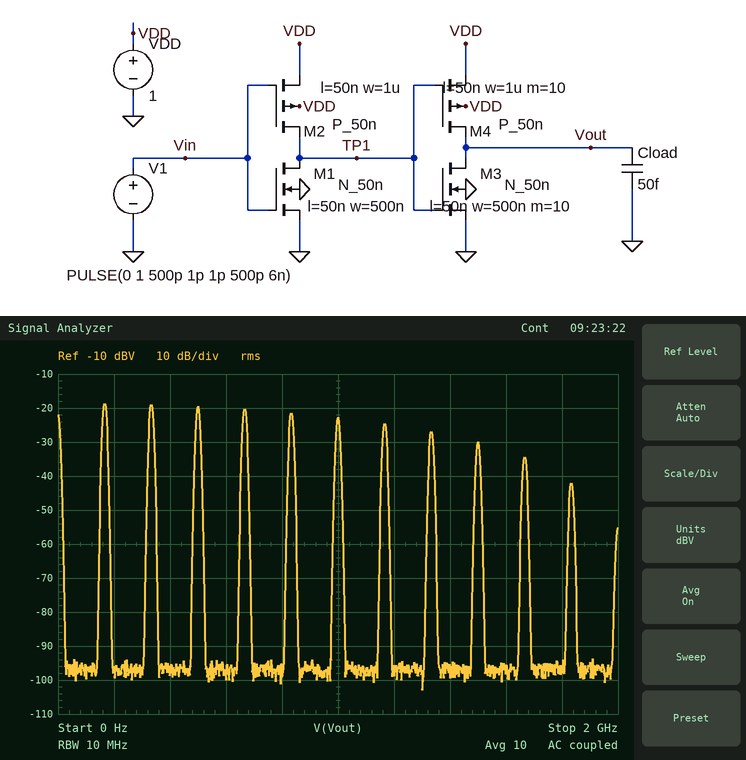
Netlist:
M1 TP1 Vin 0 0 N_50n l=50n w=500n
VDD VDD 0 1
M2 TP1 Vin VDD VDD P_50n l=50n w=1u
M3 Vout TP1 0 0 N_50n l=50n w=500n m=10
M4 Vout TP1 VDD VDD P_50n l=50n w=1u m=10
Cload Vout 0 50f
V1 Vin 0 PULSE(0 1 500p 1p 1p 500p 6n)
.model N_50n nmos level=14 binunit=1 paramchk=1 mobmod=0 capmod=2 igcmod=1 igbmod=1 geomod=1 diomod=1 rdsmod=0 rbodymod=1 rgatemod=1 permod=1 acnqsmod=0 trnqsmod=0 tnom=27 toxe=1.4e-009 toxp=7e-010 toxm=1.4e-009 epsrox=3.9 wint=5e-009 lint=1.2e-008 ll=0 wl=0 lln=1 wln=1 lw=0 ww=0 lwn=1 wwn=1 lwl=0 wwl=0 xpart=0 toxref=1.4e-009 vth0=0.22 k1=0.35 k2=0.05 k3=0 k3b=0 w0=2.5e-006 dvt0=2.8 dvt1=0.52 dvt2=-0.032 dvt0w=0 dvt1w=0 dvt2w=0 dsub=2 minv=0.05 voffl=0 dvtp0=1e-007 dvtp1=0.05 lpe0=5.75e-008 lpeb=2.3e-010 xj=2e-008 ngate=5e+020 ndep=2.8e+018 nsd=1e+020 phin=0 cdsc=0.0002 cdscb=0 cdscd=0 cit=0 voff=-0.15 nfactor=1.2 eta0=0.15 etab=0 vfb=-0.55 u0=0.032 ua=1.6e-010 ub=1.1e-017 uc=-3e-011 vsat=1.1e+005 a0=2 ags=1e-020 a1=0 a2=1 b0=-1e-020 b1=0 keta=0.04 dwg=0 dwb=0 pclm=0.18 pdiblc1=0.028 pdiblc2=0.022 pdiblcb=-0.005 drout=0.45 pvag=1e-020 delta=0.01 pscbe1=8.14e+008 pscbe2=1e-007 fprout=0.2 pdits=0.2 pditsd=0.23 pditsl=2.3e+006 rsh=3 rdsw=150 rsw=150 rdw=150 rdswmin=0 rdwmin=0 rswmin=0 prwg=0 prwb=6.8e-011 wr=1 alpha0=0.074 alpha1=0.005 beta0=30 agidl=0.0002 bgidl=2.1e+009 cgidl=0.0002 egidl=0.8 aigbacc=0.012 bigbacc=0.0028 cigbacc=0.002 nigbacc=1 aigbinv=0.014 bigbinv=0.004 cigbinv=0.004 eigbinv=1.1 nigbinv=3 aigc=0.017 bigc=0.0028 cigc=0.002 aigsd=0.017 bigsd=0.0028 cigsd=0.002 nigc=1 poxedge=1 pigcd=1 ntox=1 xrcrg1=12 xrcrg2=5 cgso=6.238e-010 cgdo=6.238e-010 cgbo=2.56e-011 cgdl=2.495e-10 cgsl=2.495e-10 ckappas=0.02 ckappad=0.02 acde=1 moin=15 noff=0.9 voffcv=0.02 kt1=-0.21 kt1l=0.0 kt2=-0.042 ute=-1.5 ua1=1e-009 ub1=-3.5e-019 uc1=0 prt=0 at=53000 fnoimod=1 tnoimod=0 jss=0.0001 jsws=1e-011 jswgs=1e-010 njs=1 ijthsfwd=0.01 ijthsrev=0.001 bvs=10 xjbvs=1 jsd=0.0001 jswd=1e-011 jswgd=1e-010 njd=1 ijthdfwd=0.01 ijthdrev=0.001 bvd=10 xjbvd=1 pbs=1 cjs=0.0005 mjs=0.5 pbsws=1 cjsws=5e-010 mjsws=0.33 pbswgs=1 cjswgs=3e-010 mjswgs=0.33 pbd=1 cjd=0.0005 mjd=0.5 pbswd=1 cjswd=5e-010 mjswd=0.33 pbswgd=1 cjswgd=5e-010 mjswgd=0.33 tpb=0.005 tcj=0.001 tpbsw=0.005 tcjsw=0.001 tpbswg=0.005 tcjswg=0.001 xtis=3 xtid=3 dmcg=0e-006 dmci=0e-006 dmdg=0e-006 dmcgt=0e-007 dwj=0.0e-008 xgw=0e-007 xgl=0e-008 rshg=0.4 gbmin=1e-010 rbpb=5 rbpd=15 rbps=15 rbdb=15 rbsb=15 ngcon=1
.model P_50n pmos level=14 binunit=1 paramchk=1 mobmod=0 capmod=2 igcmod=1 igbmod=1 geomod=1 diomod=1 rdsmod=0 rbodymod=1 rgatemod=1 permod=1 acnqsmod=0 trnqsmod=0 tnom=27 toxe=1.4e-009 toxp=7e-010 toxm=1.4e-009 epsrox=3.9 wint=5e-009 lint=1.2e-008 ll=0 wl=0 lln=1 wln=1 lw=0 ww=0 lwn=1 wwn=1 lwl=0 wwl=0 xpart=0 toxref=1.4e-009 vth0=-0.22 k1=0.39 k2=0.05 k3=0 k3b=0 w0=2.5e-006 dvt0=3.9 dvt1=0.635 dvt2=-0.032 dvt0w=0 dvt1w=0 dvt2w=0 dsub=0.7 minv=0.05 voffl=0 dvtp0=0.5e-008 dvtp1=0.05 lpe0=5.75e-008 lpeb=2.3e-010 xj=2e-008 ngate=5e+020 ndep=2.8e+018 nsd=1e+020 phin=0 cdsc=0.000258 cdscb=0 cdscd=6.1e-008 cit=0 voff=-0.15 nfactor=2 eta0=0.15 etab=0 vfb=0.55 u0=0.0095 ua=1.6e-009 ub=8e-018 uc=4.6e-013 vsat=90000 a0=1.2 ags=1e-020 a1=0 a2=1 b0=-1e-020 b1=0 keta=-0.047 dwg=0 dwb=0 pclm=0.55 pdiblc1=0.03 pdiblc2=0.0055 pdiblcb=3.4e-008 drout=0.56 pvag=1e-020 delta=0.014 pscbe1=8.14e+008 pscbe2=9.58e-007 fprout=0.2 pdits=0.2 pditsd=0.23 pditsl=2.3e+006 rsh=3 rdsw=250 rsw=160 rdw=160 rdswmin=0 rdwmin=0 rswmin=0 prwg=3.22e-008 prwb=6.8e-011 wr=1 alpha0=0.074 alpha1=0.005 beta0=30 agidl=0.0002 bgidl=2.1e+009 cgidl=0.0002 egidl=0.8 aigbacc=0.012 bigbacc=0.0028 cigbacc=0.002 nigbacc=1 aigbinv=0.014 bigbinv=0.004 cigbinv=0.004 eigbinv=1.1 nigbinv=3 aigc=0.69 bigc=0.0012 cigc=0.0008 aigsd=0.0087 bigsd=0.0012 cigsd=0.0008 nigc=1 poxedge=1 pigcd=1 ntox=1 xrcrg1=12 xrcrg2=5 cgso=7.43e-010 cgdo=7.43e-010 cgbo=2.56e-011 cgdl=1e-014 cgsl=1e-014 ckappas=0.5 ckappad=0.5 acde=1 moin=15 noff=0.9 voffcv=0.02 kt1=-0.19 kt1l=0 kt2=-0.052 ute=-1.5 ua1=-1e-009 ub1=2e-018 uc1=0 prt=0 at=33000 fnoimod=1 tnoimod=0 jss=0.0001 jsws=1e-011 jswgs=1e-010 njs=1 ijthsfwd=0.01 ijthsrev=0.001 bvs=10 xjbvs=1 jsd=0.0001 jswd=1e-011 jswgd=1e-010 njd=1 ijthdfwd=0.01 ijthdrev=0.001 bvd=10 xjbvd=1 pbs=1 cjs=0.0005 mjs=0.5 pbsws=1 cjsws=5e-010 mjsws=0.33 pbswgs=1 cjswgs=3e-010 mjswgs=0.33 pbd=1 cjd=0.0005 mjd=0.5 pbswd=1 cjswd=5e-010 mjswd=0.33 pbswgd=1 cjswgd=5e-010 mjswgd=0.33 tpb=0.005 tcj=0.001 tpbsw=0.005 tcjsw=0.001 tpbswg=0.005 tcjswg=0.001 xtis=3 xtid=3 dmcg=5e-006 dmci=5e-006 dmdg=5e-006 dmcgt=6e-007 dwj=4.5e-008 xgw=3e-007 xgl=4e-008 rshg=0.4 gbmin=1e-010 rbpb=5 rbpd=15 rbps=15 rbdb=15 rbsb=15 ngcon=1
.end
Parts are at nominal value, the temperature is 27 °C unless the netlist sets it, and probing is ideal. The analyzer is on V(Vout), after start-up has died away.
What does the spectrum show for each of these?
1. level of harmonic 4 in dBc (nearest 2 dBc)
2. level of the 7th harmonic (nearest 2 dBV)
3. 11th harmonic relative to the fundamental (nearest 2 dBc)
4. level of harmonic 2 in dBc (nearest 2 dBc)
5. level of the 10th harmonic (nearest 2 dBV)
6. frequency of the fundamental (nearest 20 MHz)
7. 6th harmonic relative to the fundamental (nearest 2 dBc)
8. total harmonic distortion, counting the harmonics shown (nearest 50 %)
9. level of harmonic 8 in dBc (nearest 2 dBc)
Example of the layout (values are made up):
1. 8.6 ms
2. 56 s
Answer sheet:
1. -2 dBc
2. -24 dBV
3. -24 dBc
4. 0 dBc
5. -34 dBV
6. 160 MHz
7. -4 dBc
8. 200 %
9. -8 dBc
